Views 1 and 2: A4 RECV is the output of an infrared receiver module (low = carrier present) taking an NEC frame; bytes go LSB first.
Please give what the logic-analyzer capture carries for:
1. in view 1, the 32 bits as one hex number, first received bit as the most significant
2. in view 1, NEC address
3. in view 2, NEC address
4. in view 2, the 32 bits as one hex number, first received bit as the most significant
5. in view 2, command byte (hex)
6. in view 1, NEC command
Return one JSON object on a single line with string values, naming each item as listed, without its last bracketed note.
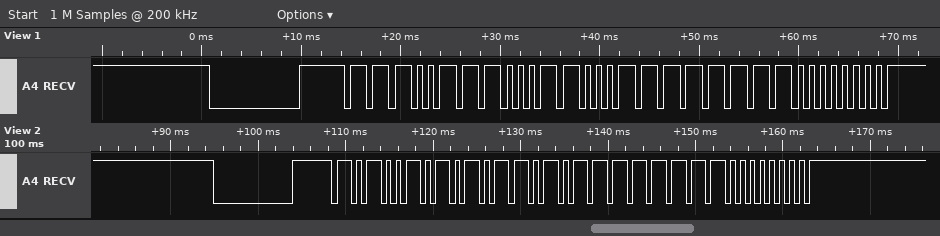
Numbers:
{"in view 1, the 32 bits as one hex number, first received bit as the most significant": "0xE718FF00", "in view 1, NEC address": "0xE7", "in view 2, NEC address": "0xA5", "in view 2, the 32 bits as one hex number, first received bit as the most significant": "0xA55AFF00", "in view 2, command byte": "0xFF", "in view 1, NEC command": "0xFF"}
